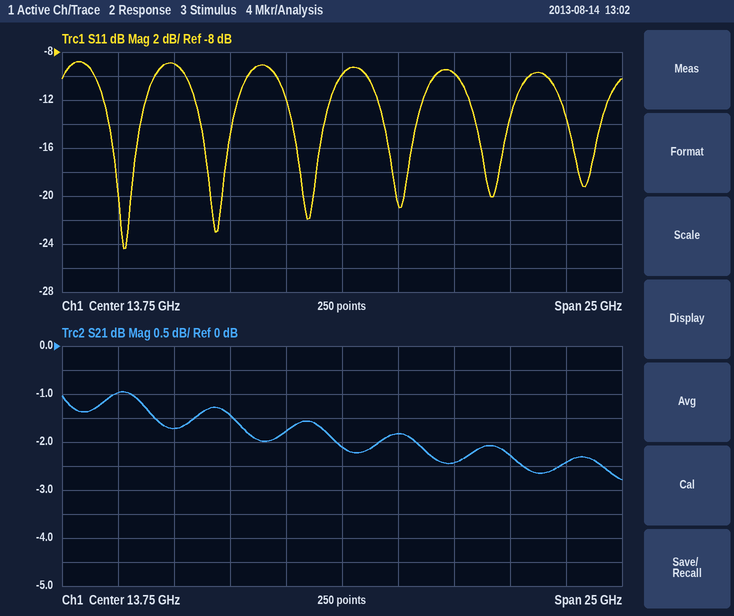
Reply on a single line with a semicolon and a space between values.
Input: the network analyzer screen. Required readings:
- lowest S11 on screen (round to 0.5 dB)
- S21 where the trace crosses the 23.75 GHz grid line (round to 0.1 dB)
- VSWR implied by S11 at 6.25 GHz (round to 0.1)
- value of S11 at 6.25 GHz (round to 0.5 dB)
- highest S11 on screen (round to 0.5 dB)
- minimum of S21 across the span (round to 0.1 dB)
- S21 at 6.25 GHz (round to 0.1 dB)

-24.5 dB; -2.4 dB; 2.1; -9.0 dB; -9.0 dB; -2.8 dB; -1.7 dB
